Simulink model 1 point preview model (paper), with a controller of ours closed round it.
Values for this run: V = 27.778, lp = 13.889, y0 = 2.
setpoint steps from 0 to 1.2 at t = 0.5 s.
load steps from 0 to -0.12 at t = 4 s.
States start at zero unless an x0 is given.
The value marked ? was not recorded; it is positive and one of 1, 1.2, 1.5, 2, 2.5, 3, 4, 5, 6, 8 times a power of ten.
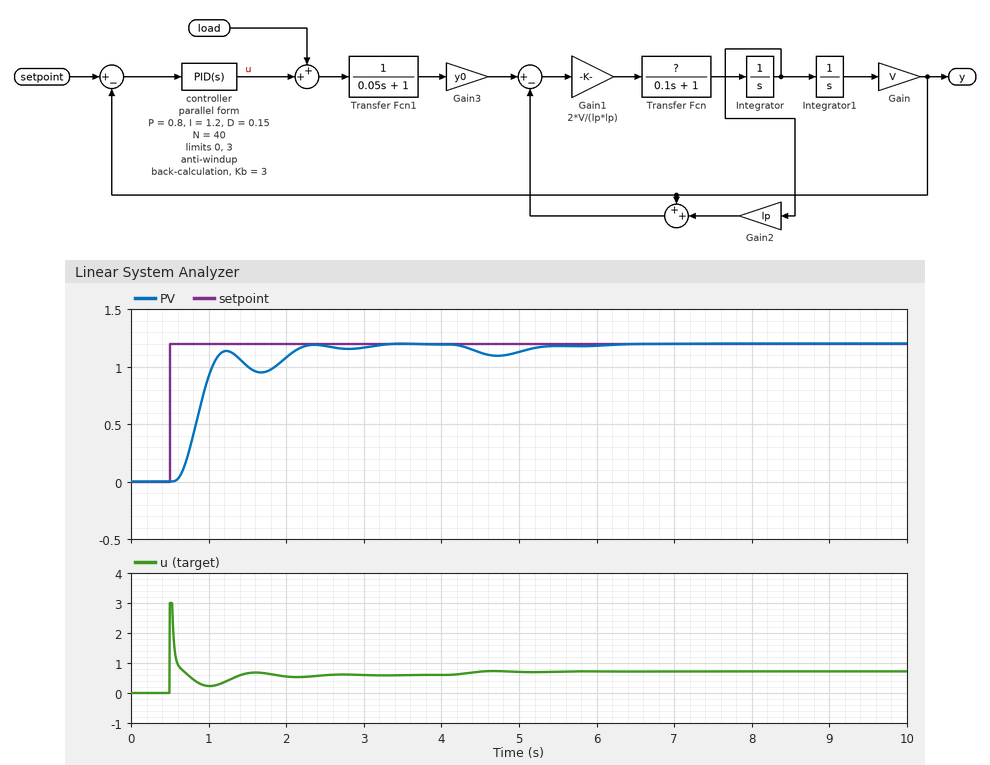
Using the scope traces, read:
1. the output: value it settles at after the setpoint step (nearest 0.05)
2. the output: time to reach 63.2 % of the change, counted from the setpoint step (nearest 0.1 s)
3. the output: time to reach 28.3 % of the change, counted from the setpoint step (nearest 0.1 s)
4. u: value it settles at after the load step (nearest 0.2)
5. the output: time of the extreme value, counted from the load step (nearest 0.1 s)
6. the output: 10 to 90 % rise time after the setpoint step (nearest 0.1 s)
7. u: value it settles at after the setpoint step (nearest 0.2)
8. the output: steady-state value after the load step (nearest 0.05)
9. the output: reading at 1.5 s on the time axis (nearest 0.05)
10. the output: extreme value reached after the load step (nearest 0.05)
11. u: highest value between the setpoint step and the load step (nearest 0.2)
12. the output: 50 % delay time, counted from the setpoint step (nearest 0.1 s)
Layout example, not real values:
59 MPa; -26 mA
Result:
1.20; 0.4 s; 0.3 s; 0.8; 0.7 s; 0.4 s; 0.6; 1.20; 1.00; 1.10; 3.0; 0.4 s
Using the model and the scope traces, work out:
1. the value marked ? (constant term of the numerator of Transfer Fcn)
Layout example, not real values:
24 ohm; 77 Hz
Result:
1
